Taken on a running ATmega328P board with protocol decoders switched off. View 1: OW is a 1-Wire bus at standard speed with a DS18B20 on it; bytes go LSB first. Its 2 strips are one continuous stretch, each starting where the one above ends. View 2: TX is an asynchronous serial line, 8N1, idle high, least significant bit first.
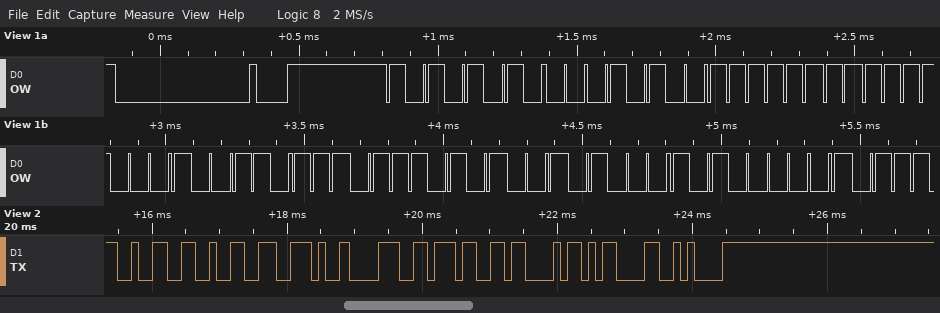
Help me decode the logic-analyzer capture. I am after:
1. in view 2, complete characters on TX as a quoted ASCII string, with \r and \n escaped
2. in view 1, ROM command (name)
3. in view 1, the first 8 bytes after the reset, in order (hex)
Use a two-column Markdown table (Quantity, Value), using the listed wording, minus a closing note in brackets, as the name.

| Quantity | Value |
|---|---|
| in view 2, complete characters on TX as a quoted ASCII string, with \r and \n escaped | "22.87C\r\n" |
| in view 1, ROM command | Match ROM |
| in view 1, the first 8 bytes after the reset, in order | 55 28 FF 8F EC AE 14 05 |
